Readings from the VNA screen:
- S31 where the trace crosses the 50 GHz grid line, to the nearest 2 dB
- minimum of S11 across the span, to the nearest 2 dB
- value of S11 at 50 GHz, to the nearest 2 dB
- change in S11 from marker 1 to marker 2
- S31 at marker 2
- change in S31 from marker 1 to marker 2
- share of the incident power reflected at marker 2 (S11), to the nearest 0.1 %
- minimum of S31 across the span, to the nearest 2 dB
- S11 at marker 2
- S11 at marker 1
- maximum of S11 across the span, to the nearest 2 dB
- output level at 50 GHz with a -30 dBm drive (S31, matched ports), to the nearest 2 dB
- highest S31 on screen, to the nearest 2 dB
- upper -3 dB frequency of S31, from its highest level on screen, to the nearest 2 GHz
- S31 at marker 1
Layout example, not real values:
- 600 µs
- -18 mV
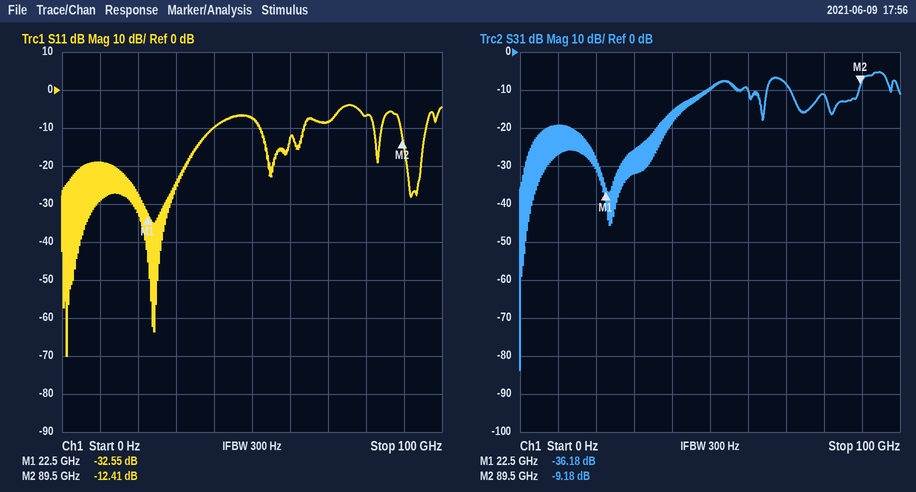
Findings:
- -10 dB
- -70 dB
- -8 dB
- 20.14 dB
- -9.18 dB
- 27.00 dB
- 5.7 %
- -84 dB
- -12.41 dB
- -32.55 dB
- -4 dB
- -40 dBm
- -6 dB
- 96 GHz
- -36.18 dB
